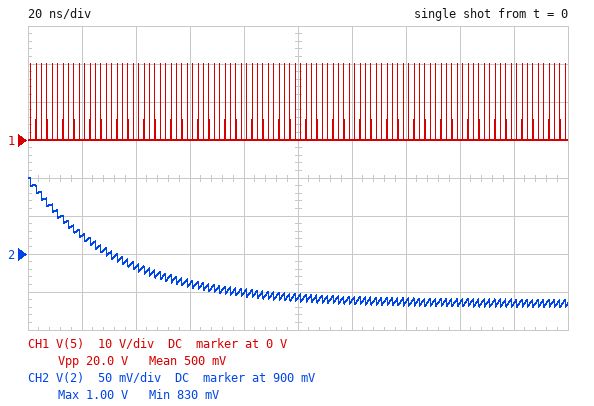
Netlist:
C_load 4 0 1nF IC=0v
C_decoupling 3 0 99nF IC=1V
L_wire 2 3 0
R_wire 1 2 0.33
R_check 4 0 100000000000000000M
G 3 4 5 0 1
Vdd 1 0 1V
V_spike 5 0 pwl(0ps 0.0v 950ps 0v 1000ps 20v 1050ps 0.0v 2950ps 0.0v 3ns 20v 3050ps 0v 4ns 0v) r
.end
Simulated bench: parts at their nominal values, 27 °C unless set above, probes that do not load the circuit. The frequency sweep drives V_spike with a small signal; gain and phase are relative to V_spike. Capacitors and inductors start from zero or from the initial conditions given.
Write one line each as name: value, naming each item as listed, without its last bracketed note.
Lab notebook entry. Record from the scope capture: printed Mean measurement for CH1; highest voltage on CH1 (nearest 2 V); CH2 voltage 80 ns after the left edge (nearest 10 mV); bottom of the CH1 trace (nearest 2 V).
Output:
printed Mean measurement for CH1: 500 mV
highest voltage on CH1: 20 V
CH2 voltage 80 ns after the left edge: 850 mV
bottom of the CH1 trace: 0 V
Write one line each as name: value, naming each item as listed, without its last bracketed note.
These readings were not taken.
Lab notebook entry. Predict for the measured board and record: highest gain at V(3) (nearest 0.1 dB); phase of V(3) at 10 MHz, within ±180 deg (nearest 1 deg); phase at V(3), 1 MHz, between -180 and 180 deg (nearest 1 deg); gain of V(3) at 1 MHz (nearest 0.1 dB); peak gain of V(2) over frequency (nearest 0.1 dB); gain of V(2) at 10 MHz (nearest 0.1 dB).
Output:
highest gain at V(3): -9.6 dB
phase of V(3) at 10 MHz, within ±180 deg: 116 deg
phase at V(3), 1 MHz, between -180 and 180 deg: 168 deg
gain of V(3) at 1 MHz: -9.8 dB
peak gain of V(2) over frequency: -9.6 dB
gain of V(2) at 10 MHz: -16.8 dB
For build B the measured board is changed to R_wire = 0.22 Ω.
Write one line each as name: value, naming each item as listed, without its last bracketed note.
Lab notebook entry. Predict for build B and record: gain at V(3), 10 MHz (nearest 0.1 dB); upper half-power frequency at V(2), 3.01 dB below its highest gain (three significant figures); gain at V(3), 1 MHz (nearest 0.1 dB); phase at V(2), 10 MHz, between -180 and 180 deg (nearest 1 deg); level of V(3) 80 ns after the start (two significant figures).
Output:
gain at V(3), 10 MHz: -17.7 dB
upper half-power frequency at V(2), 3.01 dB below its highest gain: 7.31 MHz
gain at V(3), 1 MHz: -13.2 dB
phase at V(2), 10 MHz, between -180 and 180 deg: 126 deg
level of V(3) 80 ns after the start: 890 mV
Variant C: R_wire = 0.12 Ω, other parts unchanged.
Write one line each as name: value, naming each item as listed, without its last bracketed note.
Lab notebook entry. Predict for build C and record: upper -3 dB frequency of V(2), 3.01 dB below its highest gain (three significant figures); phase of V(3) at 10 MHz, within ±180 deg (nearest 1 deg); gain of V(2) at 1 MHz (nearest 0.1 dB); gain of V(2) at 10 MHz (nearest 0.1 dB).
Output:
upper -3 dB frequency of V(2), 3.01 dB below its highest gain: 13.4 MHz
phase of V(3) at 10 MHz, within ±180 deg: 143 deg
gain of V(2) at 1 MHz: -18.4 dB
gain of V(2) at 10 MHz: -20.3 dB
